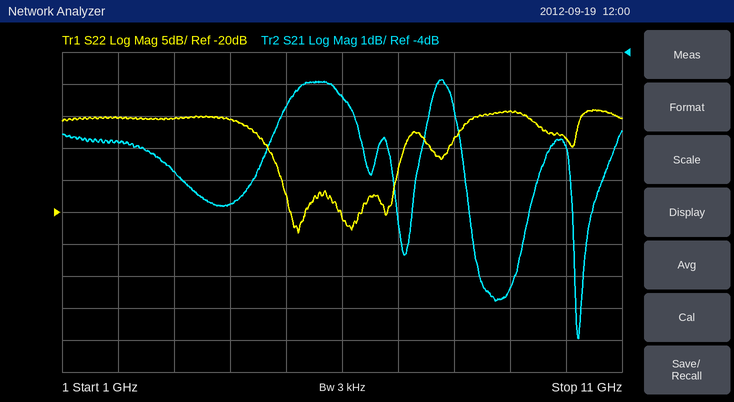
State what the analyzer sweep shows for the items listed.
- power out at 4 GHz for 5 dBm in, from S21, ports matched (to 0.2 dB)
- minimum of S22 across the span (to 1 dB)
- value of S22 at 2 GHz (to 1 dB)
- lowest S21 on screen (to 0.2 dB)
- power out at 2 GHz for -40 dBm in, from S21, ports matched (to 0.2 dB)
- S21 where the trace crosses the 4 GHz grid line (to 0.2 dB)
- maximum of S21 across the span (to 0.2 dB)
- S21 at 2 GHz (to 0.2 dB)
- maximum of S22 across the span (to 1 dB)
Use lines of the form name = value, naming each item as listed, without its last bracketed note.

power out at 4 GHz for 5 dBm in, from S21, ports matched = -3.8 dBm
minimum of S22 across the span = -23 dB
value of S22 at 2 GHz = -5 dB
lowest S21 on screen = -13.0 dB
power out at 2 GHz for -40 dBm in, from S21, ports matched = -46.8 dBm
S21 where the trace crosses the 4 GHz grid line = -8.8 dB
maximum of S21 across the span = -4.8 dB
S21 at 2 GHz = -6.8 dB
maximum of S22 across the span = -4 dB
